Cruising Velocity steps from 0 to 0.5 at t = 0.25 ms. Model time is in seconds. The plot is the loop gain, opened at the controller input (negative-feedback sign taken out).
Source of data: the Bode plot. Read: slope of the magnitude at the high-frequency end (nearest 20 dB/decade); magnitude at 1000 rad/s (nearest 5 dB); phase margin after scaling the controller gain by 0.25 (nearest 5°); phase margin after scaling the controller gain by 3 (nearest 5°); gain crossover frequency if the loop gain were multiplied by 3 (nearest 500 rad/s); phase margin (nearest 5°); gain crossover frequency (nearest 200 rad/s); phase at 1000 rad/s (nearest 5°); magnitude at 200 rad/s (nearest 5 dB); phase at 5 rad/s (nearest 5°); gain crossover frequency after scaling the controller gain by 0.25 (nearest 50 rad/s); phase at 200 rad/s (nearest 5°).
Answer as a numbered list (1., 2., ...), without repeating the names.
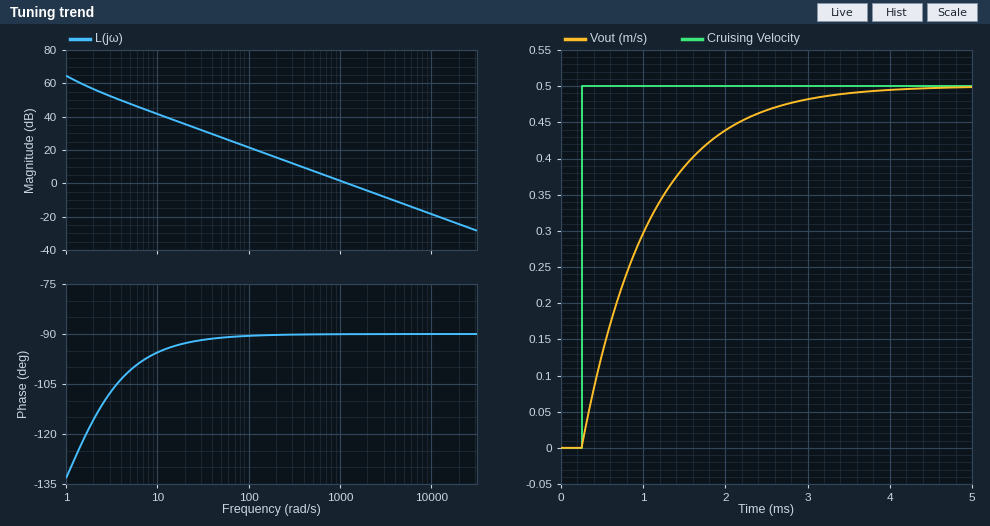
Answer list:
1. -20 dB/decade
2. 0 dB
3. 90°
4. 90°
5. 3500 rad/s
6. 90°
7. 1200 rad/s
8. -90°
9. 15 dB
10. -100°
11. 300 rad/s
12. -90°
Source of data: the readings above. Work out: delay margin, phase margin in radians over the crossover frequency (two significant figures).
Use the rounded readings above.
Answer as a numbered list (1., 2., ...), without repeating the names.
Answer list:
1. 0.0013 s
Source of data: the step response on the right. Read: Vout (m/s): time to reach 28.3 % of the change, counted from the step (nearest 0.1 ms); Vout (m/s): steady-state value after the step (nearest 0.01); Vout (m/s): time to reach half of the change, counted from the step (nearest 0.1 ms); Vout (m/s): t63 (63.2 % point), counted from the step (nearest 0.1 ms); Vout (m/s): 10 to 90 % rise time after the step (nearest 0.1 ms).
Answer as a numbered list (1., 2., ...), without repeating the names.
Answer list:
1. 0.3 ms
2. 0.50
3. 0.6 ms
4. 0.8 ms
5. 1.8 ms
